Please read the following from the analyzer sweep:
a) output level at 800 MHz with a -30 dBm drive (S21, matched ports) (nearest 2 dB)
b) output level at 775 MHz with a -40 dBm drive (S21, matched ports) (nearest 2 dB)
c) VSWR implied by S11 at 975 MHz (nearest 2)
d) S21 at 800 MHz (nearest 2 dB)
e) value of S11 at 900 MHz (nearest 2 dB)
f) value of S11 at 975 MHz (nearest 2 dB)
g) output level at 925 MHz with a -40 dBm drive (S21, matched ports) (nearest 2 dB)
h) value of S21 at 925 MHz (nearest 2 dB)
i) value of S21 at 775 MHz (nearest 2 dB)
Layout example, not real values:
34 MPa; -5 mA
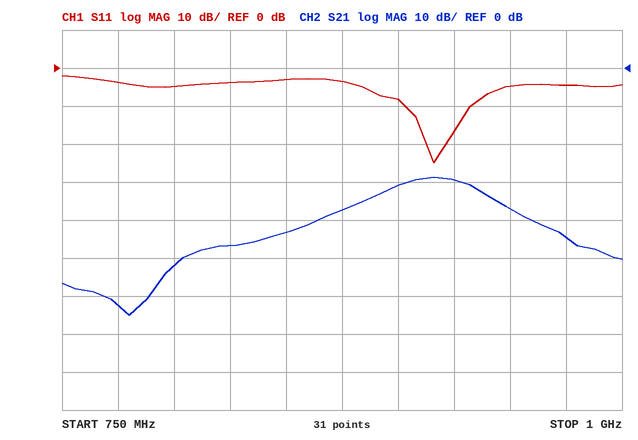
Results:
-82 dBm; -102 dBm; 4; -52 dB; -8 dB; -4 dB; -70 dBm; -30 dB; -62 dB
